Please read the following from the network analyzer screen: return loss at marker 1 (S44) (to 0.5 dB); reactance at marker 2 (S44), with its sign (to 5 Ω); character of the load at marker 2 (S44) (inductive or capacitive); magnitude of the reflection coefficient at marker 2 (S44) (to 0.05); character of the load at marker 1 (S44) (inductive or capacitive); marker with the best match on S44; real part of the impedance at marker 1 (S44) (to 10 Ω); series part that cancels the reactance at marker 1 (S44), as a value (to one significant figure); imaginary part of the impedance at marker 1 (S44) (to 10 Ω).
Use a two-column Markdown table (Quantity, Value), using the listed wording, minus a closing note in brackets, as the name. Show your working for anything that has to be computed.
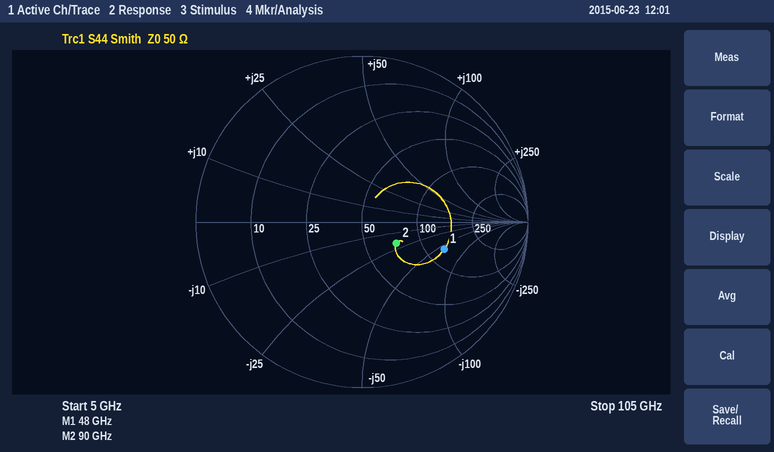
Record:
| Quantity | Value |
|---|---|
| return loss at marker 1 (S44) | 5.5 dB |
| reactance at marker 2 (S44), with its sign | -20 Ω |
| character of the load at marker 2 (S44) | capacitive |
| magnitude of the reflection coefficient at marker 2 (S44) | 0.25 |
| character of the load at marker 1 (S44) | capacitive |
| marker with the best match on S44 | marker 2 |
| real part of the impedance at marker 1 (S44) | 130 Ω |
| series part that cancels the reactance at marker 1 (S44), as a value | L = 60 Ω/(2π × 48 GHz) ≈ 199 pH, so 200 pH to one significant figure |
| imaginary part of the impedance at marker 1 (S44) | -60 Ω |
